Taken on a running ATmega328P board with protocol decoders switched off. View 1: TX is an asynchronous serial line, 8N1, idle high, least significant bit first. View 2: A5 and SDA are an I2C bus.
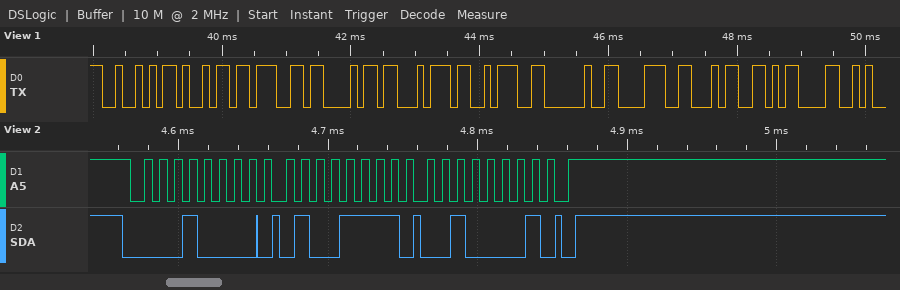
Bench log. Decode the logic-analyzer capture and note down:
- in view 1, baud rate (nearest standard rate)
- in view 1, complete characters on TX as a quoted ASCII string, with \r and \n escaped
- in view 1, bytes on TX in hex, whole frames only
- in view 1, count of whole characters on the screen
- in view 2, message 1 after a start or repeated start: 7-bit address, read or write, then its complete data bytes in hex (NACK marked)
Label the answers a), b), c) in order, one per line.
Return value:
a) 9600 baud
b) "Right: 84\r"
c) 52 69 67 68 74 3A 20 38 34 0D
d) 10
e) 0x08 write: 4F 21
